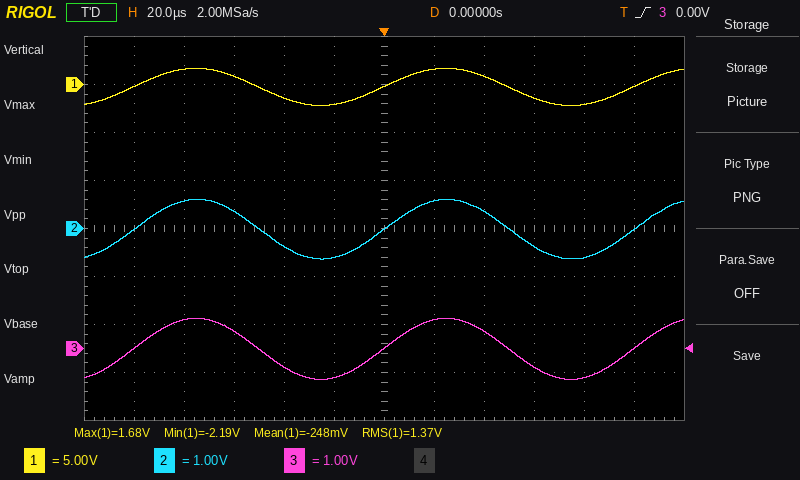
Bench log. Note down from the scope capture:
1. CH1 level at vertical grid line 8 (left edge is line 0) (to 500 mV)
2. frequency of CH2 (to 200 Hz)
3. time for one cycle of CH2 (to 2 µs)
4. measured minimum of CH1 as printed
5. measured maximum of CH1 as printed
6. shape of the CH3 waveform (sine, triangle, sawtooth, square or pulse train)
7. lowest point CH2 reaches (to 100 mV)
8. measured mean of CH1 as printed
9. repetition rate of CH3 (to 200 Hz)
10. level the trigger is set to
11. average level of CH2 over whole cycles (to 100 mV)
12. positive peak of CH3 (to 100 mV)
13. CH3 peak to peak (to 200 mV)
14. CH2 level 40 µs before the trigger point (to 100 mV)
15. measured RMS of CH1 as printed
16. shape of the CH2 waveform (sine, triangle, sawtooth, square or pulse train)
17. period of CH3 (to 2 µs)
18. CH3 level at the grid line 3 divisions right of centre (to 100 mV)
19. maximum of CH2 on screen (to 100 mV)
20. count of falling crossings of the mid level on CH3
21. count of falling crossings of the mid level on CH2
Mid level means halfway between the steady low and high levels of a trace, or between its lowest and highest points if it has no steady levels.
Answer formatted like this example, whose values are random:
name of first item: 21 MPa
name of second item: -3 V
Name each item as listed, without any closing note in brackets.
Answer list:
CH1 level at vertical grid line 8 (left edge is line 0): 1.0 V
frequency of CH2: 10.0 kHz
time for one cycle of CH2: 100 µs
measured minimum of CH1 as printed: -2.19 V
measured maximum of CH1 as printed: 1.68 V
shape of the CH3 waveform: sine
lowest point CH2 reaches: -600 mV
measured mean of CH1 as printed: -248 mV
repetition rate of CH3: 10.0 kHz
level the trigger is set to: 0.00 V
average level of CH2 over whole cycles: 0.0 V
positive peak of CH3: 600 mV
CH3 peak to peak: 1.2 V
CH2 level 40 µs before the trigger point: -400 mV
measured RMS of CH1 as printed: 1.37 V
shape of the CH2 waveform: sine
period of CH3: 100 µs
CH3 level at the grid line 3 divisions right of centre: -400 mV
maximum of CH2 on screen: 600 mV
count of falling crossings of the mid level on CH3: 2
count of falling crossings of the mid level on CH2: 2
